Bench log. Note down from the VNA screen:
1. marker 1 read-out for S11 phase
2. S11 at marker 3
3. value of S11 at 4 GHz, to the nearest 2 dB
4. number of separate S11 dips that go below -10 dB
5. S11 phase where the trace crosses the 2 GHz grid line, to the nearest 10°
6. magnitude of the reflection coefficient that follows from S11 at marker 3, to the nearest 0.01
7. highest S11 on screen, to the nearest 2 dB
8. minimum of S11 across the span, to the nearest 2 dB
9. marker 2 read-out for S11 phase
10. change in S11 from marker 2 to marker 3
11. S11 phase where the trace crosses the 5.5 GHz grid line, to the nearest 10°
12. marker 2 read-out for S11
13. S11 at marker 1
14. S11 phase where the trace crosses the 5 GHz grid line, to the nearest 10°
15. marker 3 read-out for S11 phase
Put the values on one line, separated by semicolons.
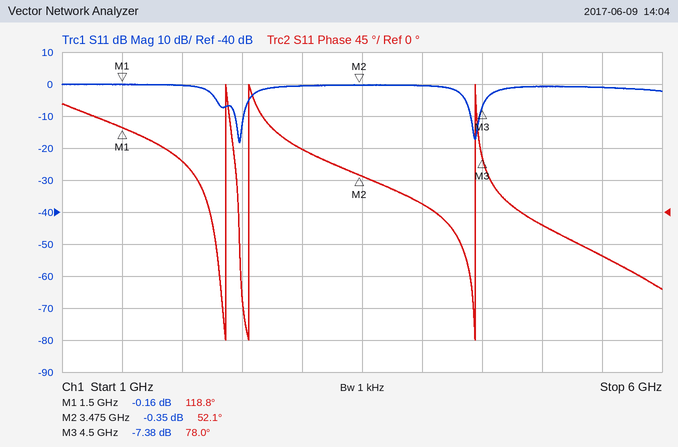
118.8°; -7.38 dB; 0 dB; 2; 70°; 0.43; 0 dB; -18 dB; 52.1°; -7.03 dB; -60°; -0.35 dB; -0.16 dB; -20°; 78.0°
